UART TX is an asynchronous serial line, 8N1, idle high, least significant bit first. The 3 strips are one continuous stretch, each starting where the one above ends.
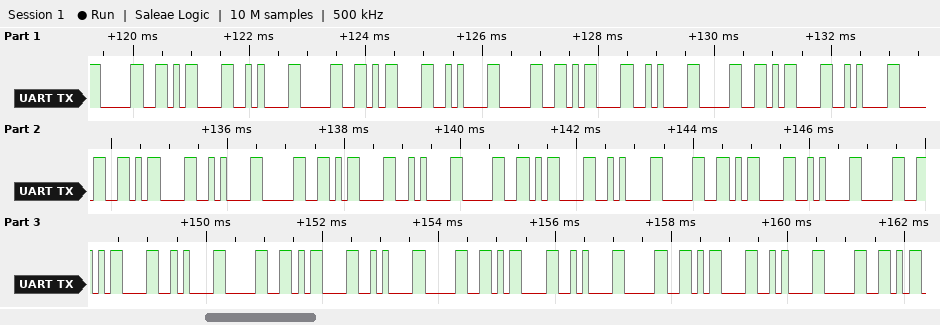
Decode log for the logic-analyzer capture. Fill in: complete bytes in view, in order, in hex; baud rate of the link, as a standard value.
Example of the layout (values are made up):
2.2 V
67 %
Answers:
30 0D 0A 30 0D 0A 30 0D 0A 30 0D 0A 30 0D 0A 30 0D 0A 30 0D 0A 30 0D 0A 30 0D 0A 30 0D 0A 30 0D 0A 30 0D 0A 30
9600 baud
